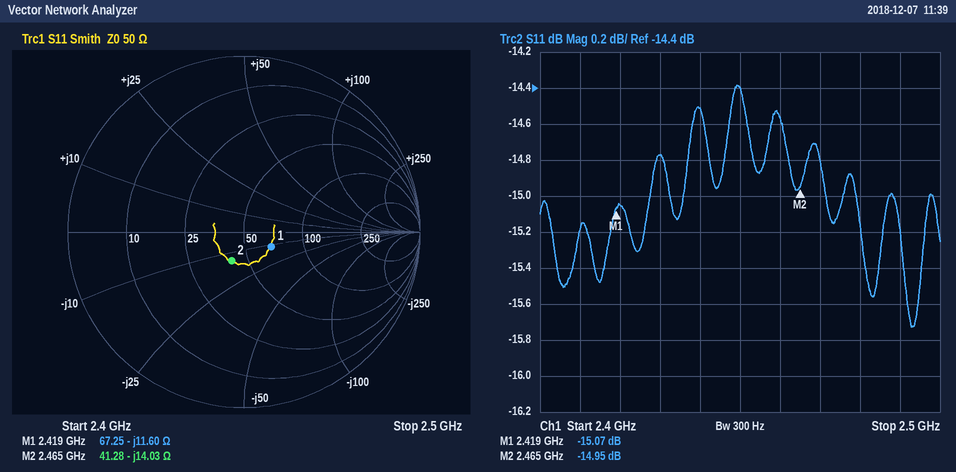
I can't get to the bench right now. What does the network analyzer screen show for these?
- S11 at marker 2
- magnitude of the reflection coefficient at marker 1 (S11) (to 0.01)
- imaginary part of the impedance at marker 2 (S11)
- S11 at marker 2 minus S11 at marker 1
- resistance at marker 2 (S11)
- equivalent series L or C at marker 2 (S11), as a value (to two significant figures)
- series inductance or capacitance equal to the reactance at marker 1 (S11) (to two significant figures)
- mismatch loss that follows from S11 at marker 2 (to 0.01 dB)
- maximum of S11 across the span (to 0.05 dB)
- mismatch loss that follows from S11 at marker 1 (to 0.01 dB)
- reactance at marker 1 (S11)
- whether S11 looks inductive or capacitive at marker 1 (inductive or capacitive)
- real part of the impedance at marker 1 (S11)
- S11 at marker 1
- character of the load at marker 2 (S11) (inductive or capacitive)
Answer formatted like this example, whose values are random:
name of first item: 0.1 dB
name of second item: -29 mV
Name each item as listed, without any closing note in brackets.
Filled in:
S11 at marker 2: -14.95 dB
magnitude of the reflection coefficient at marker 1 (S11): 0.18
imaginary part of the impedance at marker 2: -14.03 Ω
S11 at marker 2 minus S11 at marker 1: 0.12 dB
resistance at marker 2: 41.28 Ω
equivalent series L or C at marker 2 (S11), as a value: 4.6 pF
series inductance or capacitance equal to the reactance at marker 1 (S11): 5.7 pF
mismatch loss that follows from S11 at marker 2: 0.14 dB
maximum of S11 across the span: -14.40 dB
mismatch loss that follows from S11 at marker 1: 0.14 dB
reactance at marker 1: -11.60 Ω
whether S11 looks inductive or capacitive at marker 1: capacitive
real part of the impedance at marker 1: 67.25 Ω
S11 at marker 1: -15.07 dB
character of the load at marker 2 (S11): capacitive
